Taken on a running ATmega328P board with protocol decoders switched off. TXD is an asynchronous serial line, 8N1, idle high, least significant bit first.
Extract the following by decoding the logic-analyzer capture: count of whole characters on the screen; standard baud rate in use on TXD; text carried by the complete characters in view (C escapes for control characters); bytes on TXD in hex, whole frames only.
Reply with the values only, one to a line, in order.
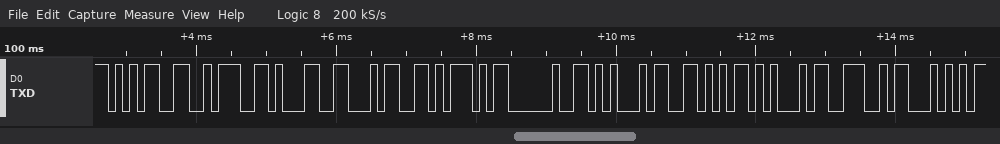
11
9600 baud
"5:14] EVENT"
0x35 0x3A 0x31 0x34 0x5D 0x20 0x45 0x56 0x45 0x4E 0x54
